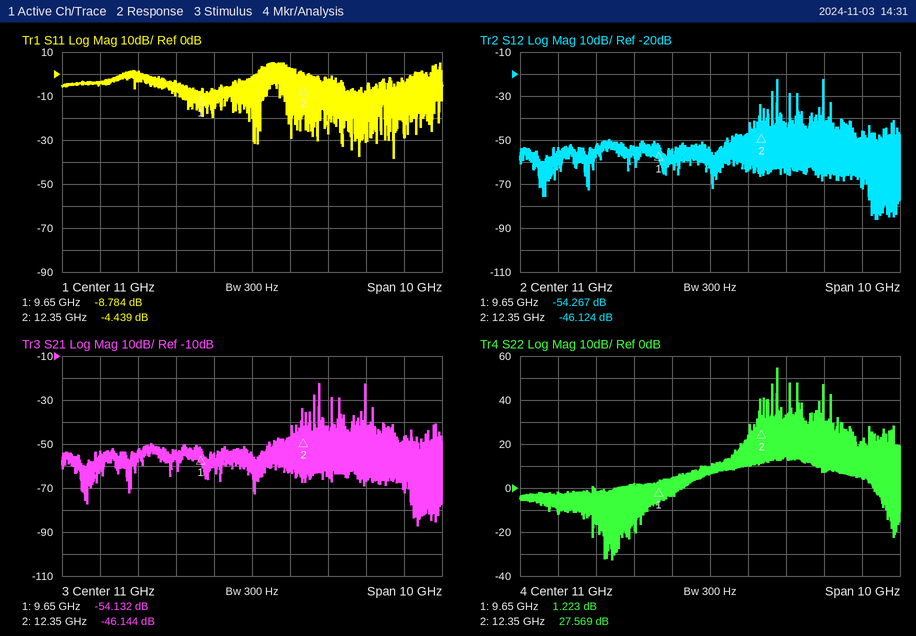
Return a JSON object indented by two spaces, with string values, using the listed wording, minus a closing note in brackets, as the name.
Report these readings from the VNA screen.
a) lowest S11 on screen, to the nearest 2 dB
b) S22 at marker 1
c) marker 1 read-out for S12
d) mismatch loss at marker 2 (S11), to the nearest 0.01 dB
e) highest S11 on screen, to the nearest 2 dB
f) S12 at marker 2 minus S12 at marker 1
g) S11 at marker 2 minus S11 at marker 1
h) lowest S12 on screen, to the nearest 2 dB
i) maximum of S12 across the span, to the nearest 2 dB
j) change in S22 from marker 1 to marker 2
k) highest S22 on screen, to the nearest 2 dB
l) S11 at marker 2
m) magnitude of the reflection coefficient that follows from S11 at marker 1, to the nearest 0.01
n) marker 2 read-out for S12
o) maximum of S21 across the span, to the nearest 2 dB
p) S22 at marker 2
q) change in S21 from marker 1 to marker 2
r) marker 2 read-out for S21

{
  "lowest S11 on screen, to the nearest 2 dB": "-38 dB",
  "S22 at marker 1": "1.223 dB",
  "marker 1 read-out for S12": "-54.267 dB",
  "mismatch loss at marker 2 (S11), to the nearest 0.01 dB": "1.94 dB",
  "highest S11 on screen, to the nearest 2 dB": "6 dB",
  "S12 at marker 2 minus S12 at marker 1": "8.143 dB",
  "S11 at marker 2 minus S11 at marker 1": "4.345 dB",
  "lowest S12 on screen, to the nearest 2 dB": "-86 dB",
  "maximum of S12 across the span, to the nearest 2 dB": "-22 dB",
  "change in S22 from marker 1 to marker 2": "26.346 dB",
  "highest S22 on screen, to the nearest 2 dB": "54 dB",
  "S11 at marker 2": "-4.439 dB",
  "magnitude of the reflection coefficient that follows from S11 at marker 1, to the nearest 0.01": "0.36",
  "marker 2 read-out for S12": "-46.124 dB",
  "maximum of S21 across the span, to the nearest 2 dB": "-22 dB",
  "S22 at marker 2": "27.569 dB",
  "change in S21 from marker 1 to marker 2": "7.988 dB",
  "marker 2 read-out for S21": "-46.144 dB"
}
